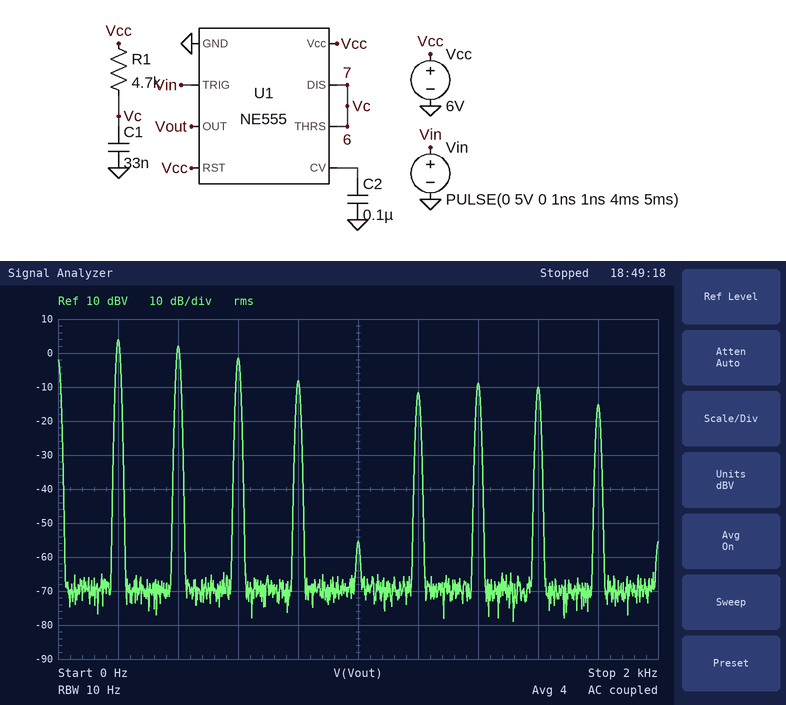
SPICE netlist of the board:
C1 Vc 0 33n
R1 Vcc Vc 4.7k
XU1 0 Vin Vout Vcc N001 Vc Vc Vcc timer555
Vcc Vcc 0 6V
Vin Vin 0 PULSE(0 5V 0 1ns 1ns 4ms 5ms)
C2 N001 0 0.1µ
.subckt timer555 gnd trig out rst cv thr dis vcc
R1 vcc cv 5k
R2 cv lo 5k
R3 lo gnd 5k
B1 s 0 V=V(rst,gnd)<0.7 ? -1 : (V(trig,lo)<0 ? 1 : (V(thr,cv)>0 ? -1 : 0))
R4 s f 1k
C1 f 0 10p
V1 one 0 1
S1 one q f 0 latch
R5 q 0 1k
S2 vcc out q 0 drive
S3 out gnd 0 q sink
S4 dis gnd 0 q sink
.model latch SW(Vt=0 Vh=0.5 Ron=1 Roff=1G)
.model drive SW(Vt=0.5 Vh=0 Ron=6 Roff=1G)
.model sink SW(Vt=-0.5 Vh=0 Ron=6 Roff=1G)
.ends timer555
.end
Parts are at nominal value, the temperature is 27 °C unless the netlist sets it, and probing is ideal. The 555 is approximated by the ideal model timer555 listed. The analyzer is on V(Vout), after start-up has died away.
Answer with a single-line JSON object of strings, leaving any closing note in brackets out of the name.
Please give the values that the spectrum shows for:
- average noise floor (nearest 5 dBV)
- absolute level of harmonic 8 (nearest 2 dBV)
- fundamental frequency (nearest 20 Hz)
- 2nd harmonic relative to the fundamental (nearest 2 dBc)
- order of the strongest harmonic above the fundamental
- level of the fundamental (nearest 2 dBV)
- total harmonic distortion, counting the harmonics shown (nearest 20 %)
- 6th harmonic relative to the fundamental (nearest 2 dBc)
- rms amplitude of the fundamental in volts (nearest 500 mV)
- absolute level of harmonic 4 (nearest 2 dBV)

{"average noise floor": "-70 dBV", "absolute level of harmonic 8": "-10 dBV", "fundamental frequency": "200 Hz", "2nd harmonic relative to the fundamental": "-2 dBc", "order of the strongest harmonic above the fundamental": "2", "level of the fundamental": "4 dBV", "total harmonic distortion, counting the harmonics shown": "100 %", "6th harmonic relative to the fundamental": "-16 dBc", "rms amplitude of the fundamental in volts": "1.5 V", "absolute level of harmonic 4": "-8 dBV"}
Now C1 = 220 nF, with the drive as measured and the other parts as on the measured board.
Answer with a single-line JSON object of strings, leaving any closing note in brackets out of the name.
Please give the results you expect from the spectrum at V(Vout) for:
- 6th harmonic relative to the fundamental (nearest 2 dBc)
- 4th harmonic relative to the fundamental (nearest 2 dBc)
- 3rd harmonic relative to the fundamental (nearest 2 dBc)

{"6th harmonic relative to the fundamental": "-12 dBc", "4th harmonic relative to the fundamental": "-20 dBc", "3rd harmonic relative to the fundamental": "-8 dBc"}
